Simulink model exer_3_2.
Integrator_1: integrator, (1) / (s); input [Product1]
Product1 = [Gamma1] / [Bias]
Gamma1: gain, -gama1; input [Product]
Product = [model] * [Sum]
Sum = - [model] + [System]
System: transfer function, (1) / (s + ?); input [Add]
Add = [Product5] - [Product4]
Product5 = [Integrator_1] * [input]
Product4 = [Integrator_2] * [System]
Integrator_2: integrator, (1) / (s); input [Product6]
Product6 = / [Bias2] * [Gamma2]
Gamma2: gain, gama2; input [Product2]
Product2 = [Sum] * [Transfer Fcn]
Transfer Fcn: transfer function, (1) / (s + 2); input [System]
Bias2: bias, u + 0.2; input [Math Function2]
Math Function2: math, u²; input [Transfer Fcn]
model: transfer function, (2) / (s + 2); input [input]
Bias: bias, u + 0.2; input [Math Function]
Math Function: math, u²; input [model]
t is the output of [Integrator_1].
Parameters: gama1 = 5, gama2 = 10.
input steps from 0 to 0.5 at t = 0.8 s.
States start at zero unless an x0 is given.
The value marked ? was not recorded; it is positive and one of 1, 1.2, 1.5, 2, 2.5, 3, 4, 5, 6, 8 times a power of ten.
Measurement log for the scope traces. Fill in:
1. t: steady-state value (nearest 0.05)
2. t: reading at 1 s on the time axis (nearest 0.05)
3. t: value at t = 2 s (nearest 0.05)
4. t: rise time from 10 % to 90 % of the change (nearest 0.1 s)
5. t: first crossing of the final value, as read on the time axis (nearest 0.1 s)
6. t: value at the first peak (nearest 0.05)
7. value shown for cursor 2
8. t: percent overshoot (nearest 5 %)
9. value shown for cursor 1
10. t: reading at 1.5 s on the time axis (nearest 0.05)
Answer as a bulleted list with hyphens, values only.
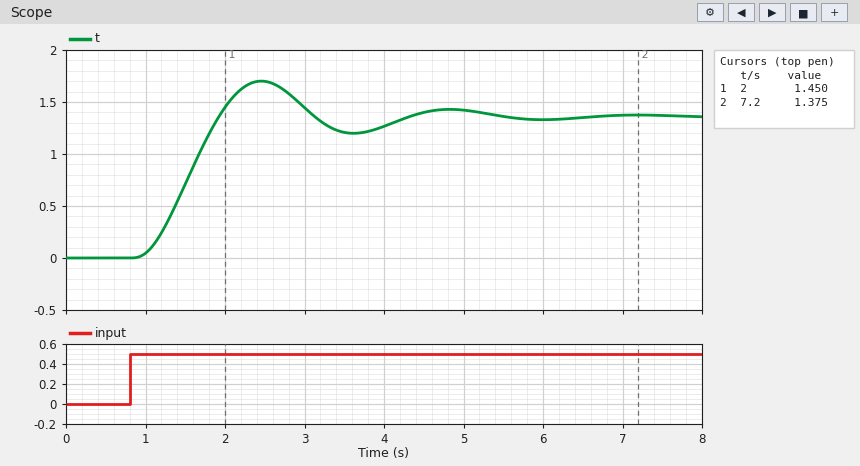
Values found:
- 1.35
- 0.05
- 1.45
- 0.7 s
- 1.9 s
- 1.70
- 1.375
- 25 %
- 1.450
- 0.70
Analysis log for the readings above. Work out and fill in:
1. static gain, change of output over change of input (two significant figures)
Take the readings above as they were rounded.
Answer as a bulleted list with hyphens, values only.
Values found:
- 2.7
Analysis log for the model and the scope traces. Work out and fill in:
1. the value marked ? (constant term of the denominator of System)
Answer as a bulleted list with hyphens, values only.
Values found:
- 1.2
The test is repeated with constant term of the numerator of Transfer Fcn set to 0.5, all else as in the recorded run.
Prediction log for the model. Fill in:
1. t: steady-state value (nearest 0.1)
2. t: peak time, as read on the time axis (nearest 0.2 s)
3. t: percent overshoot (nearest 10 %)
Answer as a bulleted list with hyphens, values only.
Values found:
- 1.4
- 2.6 s
- 30 %
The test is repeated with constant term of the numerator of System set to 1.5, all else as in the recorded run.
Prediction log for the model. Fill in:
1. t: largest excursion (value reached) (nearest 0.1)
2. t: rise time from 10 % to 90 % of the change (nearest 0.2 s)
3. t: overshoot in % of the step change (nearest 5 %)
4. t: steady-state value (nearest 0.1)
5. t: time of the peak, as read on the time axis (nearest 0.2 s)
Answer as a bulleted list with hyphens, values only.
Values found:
- 1.3
- 0.6 s
- 30 %
- 1.0
- 2.2 s
